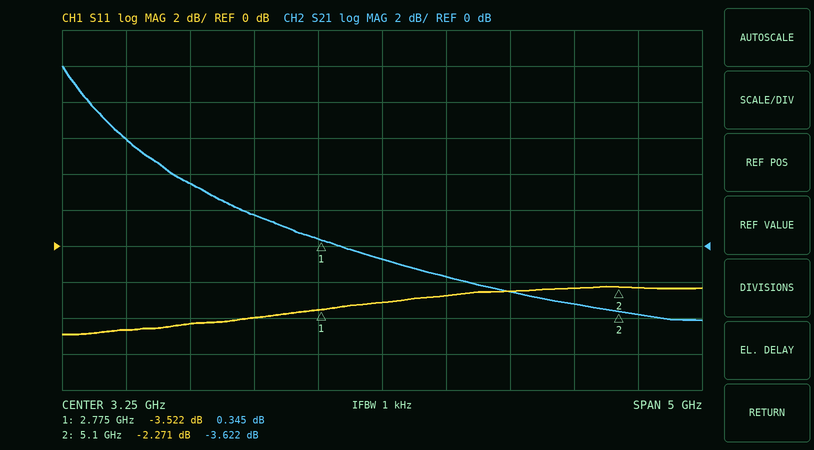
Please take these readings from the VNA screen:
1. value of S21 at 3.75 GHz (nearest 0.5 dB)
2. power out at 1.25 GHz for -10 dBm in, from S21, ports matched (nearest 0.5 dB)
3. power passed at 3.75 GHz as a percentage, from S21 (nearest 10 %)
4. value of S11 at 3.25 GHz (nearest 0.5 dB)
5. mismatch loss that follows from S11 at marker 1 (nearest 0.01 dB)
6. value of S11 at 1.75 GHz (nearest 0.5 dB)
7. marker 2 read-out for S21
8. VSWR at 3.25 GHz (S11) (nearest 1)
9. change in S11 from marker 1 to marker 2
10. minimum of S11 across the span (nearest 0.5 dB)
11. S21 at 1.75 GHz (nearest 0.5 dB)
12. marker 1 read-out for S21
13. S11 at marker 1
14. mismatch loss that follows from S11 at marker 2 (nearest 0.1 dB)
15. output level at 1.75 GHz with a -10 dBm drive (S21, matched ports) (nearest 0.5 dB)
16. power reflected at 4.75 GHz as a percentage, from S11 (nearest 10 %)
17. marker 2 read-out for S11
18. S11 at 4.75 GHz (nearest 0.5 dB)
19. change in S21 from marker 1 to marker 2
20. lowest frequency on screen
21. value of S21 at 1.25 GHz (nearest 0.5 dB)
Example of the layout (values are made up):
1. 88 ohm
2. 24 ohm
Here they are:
1. -1.5 dB
2. -4.0 dBm
3. 70 %
4. -3.0 dB
5. 2.55 dB
6. -4.5 dB
7. -3.622 dB
8. 6
9. 1.251 dB
10. -5.0 dB
11. 3.5 dB
12. 0.345 dB
13. -3.522 dB
14. 3.9 dB
15. -6.5 dBm
16. 60 %
17. -2.271 dB
18. -2.5 dB
19. -3.967 dB
20. 750 MHz
21. 6.0 dB
